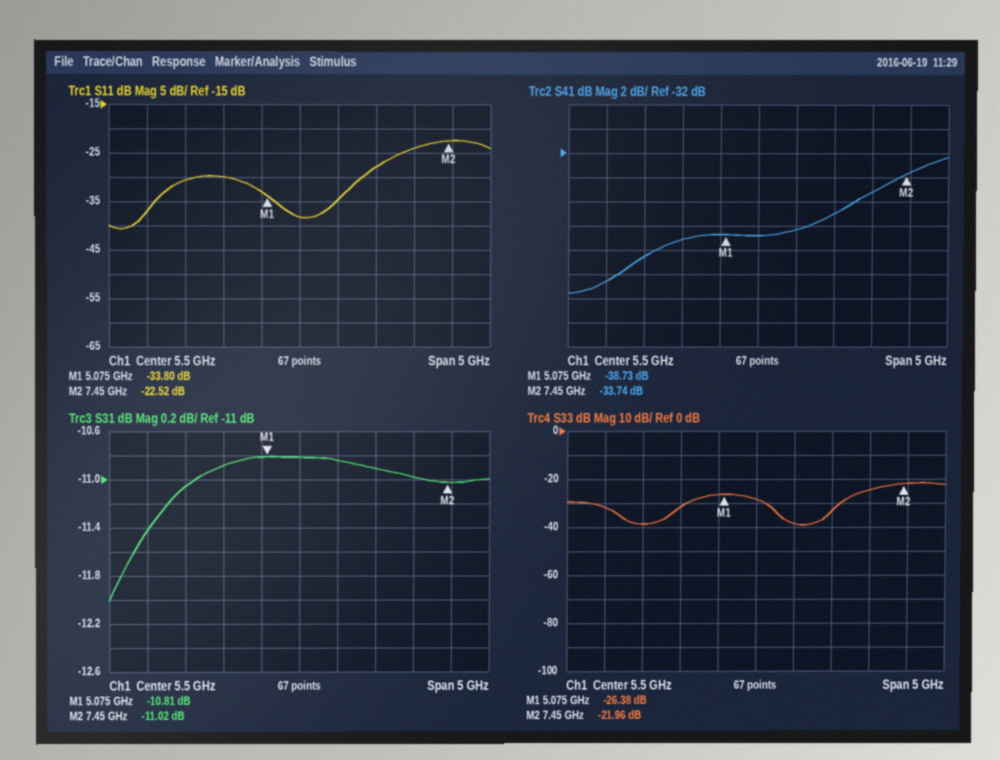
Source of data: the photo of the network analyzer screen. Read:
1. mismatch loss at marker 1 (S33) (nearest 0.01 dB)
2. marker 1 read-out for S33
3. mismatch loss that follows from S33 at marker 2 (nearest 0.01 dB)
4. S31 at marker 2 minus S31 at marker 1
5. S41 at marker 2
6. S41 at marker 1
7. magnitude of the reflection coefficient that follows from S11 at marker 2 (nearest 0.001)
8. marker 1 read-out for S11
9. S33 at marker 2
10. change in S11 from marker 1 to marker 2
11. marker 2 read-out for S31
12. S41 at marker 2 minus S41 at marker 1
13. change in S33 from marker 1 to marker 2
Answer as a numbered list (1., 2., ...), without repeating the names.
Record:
1. 0.01 dB
2. -26.38 dB
3. 0.03 dB
4. -0.21 dB
5. -33.74 dB
6. -38.73 dB
7. 0.075
8. -33.80 dB
9. -21.96 dB
10. 11.28 dB
11. -11.02 dB
12. 4.99 dB
13. 4.42 dB
